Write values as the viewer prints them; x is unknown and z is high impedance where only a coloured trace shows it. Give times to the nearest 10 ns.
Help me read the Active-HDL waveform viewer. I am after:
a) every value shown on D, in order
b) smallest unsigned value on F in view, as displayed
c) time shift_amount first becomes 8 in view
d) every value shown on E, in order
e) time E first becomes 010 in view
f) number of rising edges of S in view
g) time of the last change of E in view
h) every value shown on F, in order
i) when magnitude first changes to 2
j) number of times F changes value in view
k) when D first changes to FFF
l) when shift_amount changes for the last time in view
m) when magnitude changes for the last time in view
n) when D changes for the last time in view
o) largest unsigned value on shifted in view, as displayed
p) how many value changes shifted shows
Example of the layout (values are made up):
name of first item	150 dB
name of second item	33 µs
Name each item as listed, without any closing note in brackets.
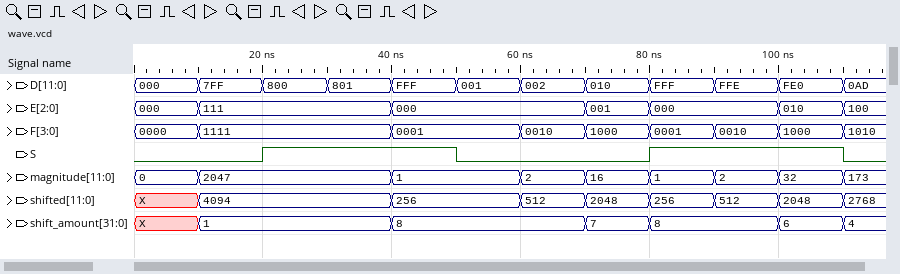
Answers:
every value shown on D, in order	000, 7FF, 800, 801, FFF, 001, 002, 010, FFF, FFE, FE0, 0AD
smallest unsigned value on F in view, as displayed	0000
time shift_amount first becomes 8 in view	40 ns
every value shown on E, in order	000, 111, 000, 001, 000, 010, 100
time E first becomes 010 in view	100 ns
number of rising edges of S in view	2
time of the last change of E in view	110 ns
every value shown on F, in order	0000, 1111, 0001, 0010, 1000, 0001, 0010, 1000, 1010
when magnitude first changes to 2	60 ns
number of times F changes value in view	8
when D first changes to FFF	40 ns
when shift_amount changes for the last time in view	110 ns
when magnitude changes for the last time in view	110 ns
when D changes for the last time in view	110 ns
largest unsigned value on shifted in view, as displayed	4094
how many value changes shifted shows	8
